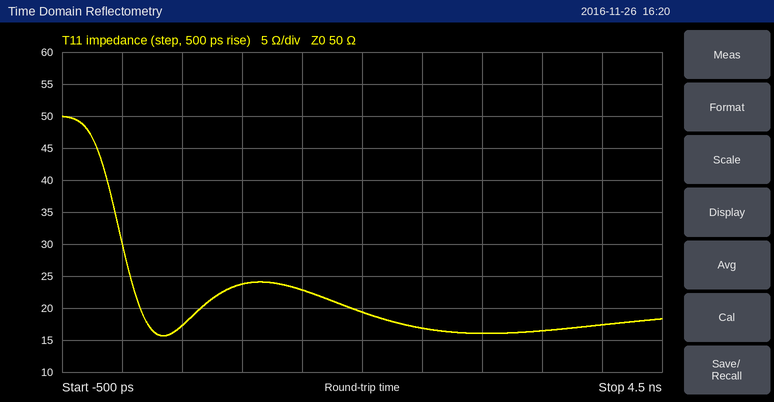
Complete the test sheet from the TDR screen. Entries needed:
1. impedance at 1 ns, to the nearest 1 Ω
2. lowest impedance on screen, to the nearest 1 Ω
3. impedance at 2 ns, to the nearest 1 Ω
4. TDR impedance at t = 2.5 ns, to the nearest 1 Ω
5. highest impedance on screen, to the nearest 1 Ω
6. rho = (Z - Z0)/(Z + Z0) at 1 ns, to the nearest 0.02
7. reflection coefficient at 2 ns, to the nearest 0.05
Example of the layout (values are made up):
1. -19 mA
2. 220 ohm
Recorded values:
1. 24 Ω
2. 16 Ω
3. 19 Ω
4. 17 Ω
5. 50 Ω
6. -0.36
7. -0.45
